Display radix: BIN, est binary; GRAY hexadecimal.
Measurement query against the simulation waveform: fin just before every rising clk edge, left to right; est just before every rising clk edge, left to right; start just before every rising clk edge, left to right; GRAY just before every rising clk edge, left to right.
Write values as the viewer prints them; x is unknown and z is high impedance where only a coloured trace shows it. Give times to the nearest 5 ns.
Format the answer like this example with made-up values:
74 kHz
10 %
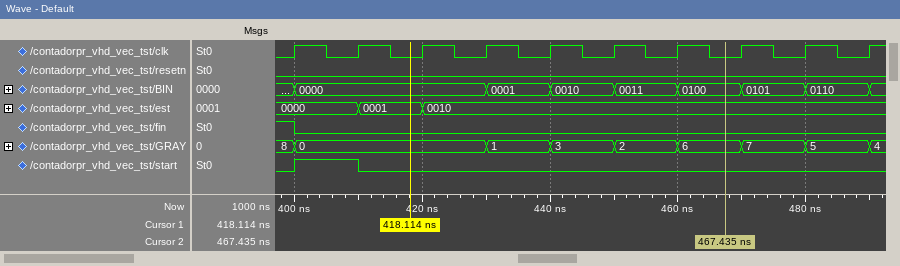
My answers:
1 0 0 0 0 0 0 0 0 0
0000, 0000, 0001, 0010, 0010, 0010, 0010, 0010, 0010, 0010
0 1 0 0 0 0 0 0 0 0
8, 0, 0, 0, 1, 3, 2, 6, 7, 5
